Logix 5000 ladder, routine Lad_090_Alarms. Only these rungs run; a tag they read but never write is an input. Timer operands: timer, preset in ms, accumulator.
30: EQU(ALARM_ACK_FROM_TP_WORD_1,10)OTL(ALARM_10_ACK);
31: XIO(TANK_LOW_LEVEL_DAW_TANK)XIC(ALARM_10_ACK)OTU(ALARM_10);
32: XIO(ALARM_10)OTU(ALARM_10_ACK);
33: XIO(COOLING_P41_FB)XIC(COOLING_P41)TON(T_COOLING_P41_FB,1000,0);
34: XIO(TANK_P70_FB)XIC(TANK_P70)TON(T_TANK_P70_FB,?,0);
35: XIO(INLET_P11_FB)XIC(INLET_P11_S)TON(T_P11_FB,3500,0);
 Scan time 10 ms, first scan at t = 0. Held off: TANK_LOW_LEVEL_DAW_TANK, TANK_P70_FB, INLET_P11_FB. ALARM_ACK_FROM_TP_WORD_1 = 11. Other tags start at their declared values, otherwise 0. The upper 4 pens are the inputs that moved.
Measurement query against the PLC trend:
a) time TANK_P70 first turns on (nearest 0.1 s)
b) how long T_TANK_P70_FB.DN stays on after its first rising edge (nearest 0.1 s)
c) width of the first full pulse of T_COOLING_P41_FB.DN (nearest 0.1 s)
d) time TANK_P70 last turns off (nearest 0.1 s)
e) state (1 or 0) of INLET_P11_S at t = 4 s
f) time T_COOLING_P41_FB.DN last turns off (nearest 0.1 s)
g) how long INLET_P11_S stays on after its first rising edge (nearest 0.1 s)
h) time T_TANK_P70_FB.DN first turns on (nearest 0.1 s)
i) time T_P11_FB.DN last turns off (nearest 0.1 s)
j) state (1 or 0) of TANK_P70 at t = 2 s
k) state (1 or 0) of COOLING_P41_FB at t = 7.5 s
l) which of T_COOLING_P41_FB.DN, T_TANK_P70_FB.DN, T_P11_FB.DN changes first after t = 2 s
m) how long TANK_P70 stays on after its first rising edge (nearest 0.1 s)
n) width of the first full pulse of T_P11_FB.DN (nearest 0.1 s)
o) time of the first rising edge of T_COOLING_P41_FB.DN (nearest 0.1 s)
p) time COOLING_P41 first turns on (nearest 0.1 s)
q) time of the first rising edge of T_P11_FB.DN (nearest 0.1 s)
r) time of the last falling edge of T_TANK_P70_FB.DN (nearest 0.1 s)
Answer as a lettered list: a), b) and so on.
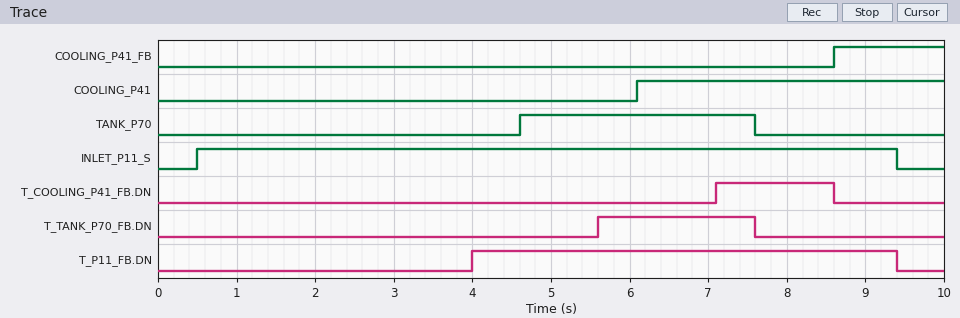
a) 4.6 s
b) 2.0 s
c) 1.5 s
d) 7.6 s
e) 1
f) 8.6 s
g) 8.9 s
h) 5.6 s
i) 9.4 s
j) 0
k) 0
l) T_P11_FB.DN
m) 3.0 s
n) 5.4 s
o) 7.1 s
p) 6.1 s
q) 4.0 s
r) 7.6 s
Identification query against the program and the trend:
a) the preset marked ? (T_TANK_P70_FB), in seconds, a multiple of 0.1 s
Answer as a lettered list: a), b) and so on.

a) 1.0 s
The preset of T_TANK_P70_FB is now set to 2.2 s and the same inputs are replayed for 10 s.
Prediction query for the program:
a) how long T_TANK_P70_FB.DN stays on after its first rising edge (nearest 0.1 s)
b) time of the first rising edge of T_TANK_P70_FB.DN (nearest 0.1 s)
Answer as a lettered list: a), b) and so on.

a) 0.8 s
b) 6.8 s
